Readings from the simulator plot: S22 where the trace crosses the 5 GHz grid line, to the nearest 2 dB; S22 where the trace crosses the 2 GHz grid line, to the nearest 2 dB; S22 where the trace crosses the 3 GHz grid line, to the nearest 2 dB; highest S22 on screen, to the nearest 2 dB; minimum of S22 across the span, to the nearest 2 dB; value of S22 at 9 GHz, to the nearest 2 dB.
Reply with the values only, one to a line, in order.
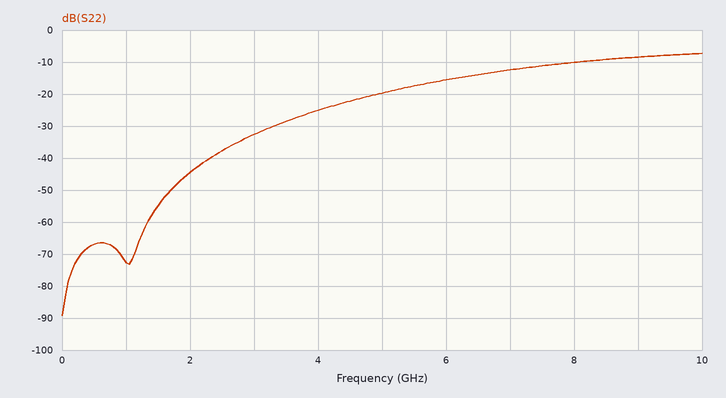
-20 dB
-44 dB
-32 dB
-8 dB
-90 dB
-8 dB
